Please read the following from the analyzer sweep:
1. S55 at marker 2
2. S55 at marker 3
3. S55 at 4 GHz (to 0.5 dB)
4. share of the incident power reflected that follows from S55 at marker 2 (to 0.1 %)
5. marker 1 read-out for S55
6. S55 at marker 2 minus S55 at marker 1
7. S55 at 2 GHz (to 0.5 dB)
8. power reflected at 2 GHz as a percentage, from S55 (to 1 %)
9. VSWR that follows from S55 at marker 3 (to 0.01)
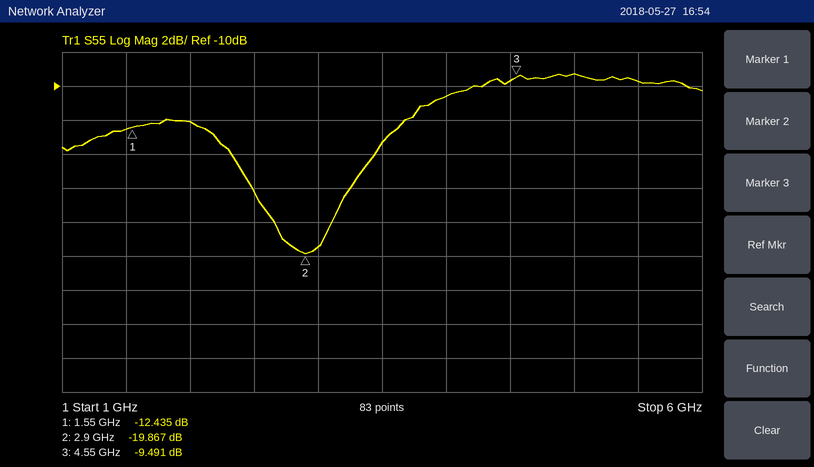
-19.867 dB
-9.491 dB
-10.5 dB
1.0 %
-12.435 dB
-7.432 dB
-12.0 dB
6 %
2.01
